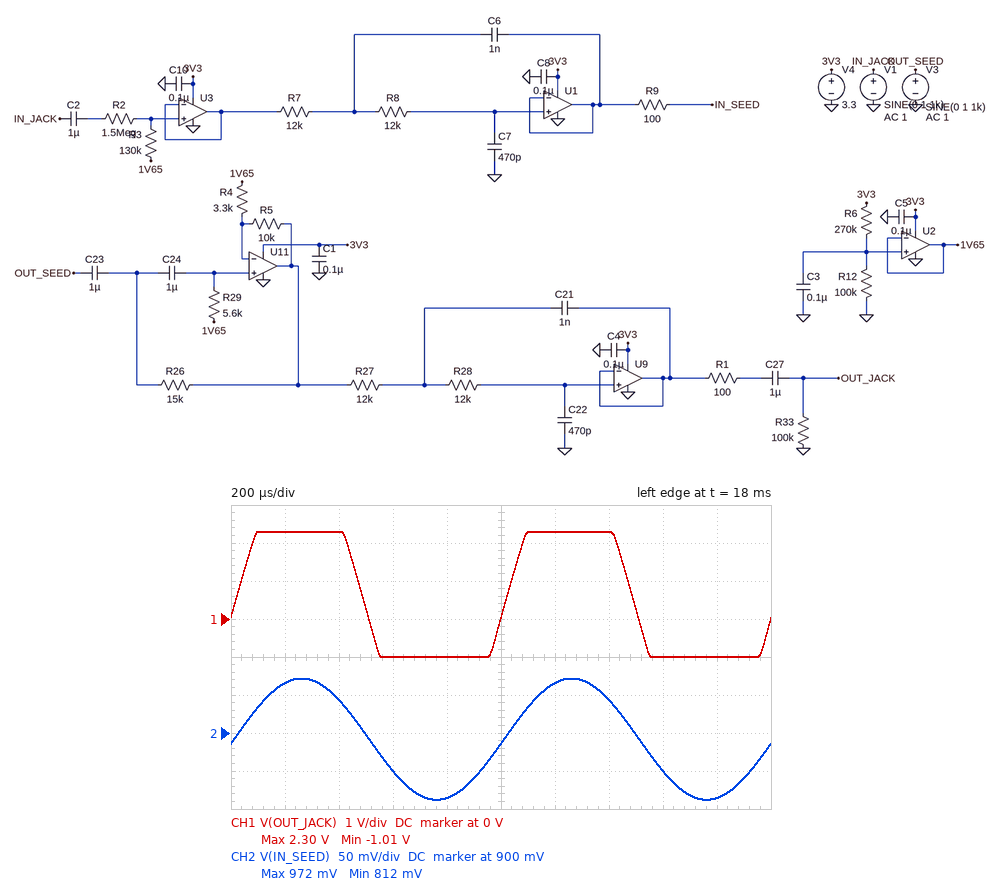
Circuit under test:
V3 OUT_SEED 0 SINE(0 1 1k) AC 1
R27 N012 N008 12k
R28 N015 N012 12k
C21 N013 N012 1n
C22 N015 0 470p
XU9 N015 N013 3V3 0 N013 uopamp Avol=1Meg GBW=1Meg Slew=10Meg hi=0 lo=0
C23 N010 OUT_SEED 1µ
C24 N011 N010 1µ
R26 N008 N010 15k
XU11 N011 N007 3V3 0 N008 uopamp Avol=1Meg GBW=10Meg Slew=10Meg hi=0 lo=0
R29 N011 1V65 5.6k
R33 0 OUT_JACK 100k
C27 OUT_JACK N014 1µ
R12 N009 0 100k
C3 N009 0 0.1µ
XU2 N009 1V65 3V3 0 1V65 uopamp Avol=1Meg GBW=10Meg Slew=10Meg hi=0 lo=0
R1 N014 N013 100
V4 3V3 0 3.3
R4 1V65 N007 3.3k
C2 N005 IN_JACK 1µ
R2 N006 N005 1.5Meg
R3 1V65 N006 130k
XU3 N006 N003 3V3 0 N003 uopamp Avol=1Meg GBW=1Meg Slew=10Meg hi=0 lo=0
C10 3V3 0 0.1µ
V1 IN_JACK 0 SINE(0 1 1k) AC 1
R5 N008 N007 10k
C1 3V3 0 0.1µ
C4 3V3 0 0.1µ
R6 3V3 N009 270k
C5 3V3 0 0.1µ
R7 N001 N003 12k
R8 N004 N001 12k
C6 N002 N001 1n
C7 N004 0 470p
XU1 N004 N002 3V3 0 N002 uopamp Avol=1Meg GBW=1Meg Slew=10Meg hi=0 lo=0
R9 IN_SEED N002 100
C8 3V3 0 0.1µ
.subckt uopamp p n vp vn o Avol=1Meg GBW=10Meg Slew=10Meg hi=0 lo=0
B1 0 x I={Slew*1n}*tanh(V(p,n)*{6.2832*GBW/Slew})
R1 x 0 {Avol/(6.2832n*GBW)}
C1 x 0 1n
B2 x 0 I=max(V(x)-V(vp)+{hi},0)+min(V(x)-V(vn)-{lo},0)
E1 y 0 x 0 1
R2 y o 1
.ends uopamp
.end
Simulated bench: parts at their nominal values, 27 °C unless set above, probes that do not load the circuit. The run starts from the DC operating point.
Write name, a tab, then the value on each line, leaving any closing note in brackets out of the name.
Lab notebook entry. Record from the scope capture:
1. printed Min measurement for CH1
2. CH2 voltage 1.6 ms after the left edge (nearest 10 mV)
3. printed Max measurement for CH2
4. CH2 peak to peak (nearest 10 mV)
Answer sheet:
printed Min measurement for CH1	-1.01 V
CH2 voltage 1.6 ms after the left edge	850 mV
printed Max measurement for CH2	972 mV
CH2 peak to peak	160 mV
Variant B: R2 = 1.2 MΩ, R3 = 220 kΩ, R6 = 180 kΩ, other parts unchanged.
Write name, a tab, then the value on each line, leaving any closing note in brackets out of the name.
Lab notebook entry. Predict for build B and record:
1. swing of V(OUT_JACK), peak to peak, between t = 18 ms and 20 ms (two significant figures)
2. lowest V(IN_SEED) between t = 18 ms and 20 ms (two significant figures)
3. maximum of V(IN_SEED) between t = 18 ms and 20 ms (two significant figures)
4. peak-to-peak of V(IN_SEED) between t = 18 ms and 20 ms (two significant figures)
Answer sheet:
swing of V(OUT_JACK), peak to peak, between t = 18 ms and 20 ms	3.3 V
lowest V(IN_SEED) between t = 18 ms and 20 ms	1.0 V
maximum of V(IN_SEED) between t = 18 ms and 20 ms	1.3 V
peak-to-peak of V(IN_SEED) between t = 18 ms and 20 ms	310 mV
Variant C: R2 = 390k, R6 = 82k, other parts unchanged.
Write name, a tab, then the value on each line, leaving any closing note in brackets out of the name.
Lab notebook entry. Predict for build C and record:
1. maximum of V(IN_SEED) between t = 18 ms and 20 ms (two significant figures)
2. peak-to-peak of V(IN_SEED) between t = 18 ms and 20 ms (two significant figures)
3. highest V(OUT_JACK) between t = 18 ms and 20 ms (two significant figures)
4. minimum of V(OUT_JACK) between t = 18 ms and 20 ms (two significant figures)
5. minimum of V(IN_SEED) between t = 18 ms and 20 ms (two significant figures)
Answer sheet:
maximum of V(IN_SEED) between t = 18 ms and 20 ms	2.1 V
peak-to-peak of V(IN_SEED) between t = 18 ms and 20 ms	500 mV
highest V(OUT_JACK) between t = 18 ms and 20 ms	1.5 V
minimum of V(OUT_JACK) between t = 18 ms and 20 ms	-1.8 V
minimum of V(IN_SEED) between t = 18 ms and 20 ms	1.6 V
